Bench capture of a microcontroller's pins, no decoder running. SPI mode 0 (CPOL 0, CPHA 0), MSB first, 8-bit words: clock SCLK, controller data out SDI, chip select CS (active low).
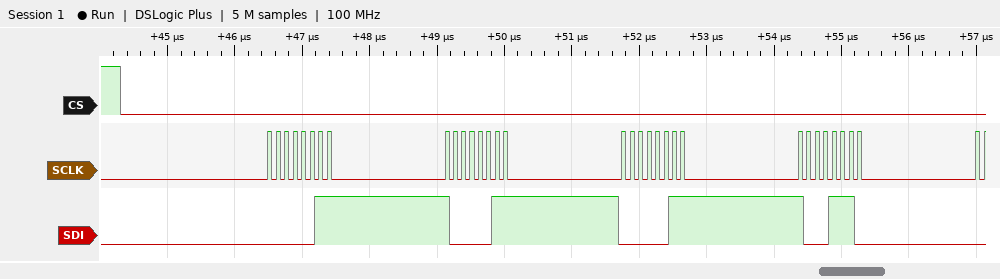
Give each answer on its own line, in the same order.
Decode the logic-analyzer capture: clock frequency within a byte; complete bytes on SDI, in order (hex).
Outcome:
8 MHz
03 83 03 8E
